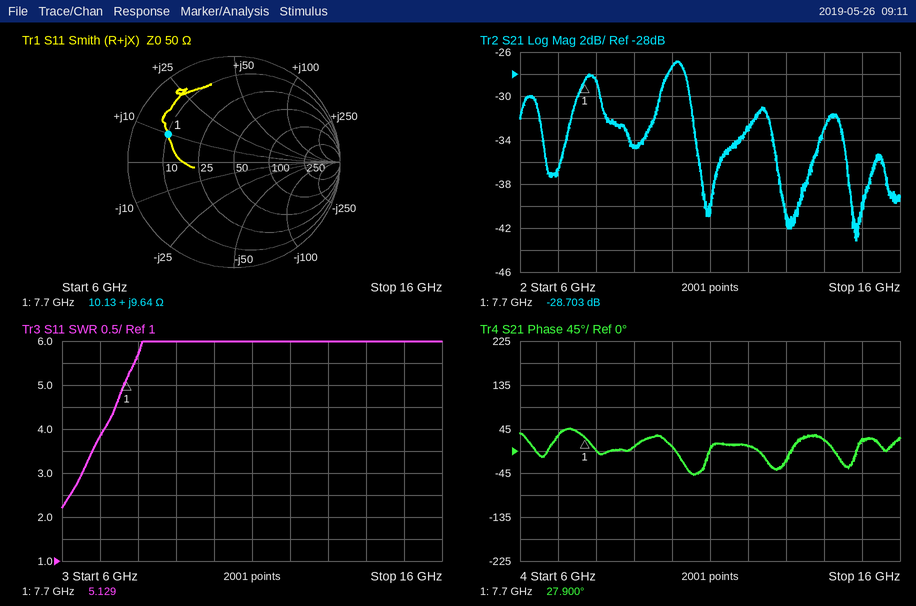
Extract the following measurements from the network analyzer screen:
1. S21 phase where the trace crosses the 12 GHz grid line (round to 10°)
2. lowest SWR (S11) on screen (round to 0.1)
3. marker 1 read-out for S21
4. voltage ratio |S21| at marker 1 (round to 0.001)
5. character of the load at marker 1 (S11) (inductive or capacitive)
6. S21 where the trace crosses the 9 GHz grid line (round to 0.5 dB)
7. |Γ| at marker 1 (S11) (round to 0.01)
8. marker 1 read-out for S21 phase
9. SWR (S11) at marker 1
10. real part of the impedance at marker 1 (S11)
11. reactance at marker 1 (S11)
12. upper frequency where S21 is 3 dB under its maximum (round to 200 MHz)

10°
2.2
-28.703 dB
0.037
inductive
-34.5 dB
0.67
27.900°
5.129
10.13 Ω
+9.64 Ω
10.4 GHz
